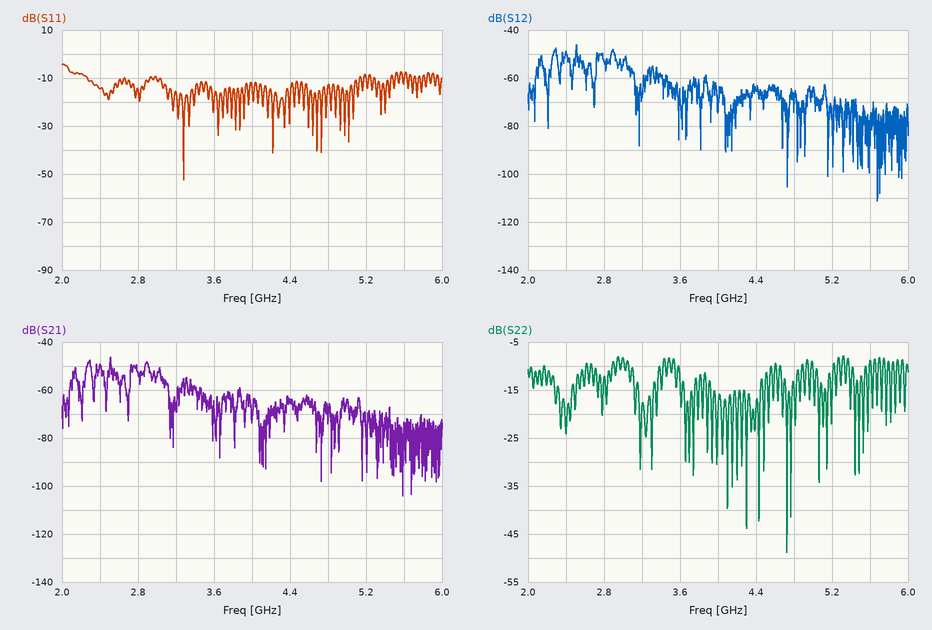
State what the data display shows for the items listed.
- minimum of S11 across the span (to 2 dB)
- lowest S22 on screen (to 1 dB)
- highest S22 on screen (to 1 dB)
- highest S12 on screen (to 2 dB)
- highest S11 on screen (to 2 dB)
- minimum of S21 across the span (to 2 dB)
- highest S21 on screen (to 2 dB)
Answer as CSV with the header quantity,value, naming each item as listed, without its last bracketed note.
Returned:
quantity,value
minimum of S11 across the span,-52 dB
lowest S22 on screen,-49 dB
highest S22 on screen,-8 dB
highest S12 on screen,-46 dB
highest S11 on screen,-4 dB
minimum of S21 across the span,-104 dB
highest S21 on screen,-46 dB
